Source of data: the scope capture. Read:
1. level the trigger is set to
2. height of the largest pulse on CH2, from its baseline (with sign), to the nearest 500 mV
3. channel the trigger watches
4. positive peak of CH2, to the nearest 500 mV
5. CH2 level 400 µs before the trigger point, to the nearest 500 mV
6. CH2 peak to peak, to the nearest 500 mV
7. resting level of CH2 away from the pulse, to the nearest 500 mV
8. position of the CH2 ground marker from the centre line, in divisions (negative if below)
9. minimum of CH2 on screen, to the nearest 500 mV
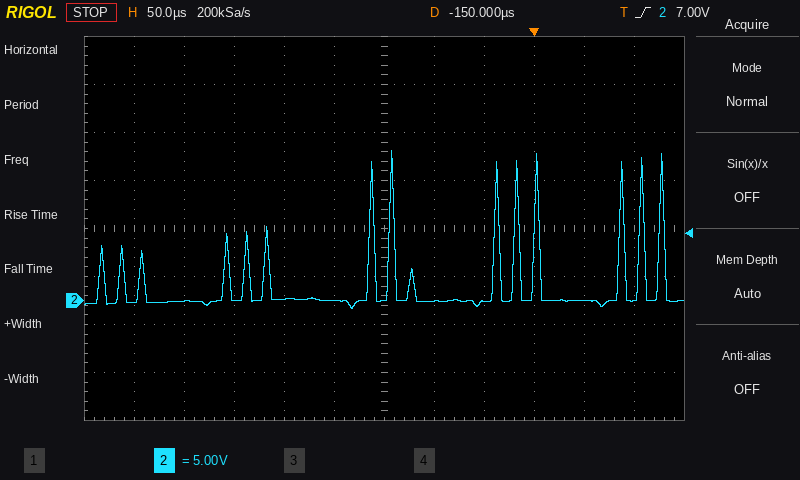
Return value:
7.00 V
+15.5 V
CH2
15.5 V
0.0 V
16.5 V
0.0 V
-1.5 div
-1.0 V
